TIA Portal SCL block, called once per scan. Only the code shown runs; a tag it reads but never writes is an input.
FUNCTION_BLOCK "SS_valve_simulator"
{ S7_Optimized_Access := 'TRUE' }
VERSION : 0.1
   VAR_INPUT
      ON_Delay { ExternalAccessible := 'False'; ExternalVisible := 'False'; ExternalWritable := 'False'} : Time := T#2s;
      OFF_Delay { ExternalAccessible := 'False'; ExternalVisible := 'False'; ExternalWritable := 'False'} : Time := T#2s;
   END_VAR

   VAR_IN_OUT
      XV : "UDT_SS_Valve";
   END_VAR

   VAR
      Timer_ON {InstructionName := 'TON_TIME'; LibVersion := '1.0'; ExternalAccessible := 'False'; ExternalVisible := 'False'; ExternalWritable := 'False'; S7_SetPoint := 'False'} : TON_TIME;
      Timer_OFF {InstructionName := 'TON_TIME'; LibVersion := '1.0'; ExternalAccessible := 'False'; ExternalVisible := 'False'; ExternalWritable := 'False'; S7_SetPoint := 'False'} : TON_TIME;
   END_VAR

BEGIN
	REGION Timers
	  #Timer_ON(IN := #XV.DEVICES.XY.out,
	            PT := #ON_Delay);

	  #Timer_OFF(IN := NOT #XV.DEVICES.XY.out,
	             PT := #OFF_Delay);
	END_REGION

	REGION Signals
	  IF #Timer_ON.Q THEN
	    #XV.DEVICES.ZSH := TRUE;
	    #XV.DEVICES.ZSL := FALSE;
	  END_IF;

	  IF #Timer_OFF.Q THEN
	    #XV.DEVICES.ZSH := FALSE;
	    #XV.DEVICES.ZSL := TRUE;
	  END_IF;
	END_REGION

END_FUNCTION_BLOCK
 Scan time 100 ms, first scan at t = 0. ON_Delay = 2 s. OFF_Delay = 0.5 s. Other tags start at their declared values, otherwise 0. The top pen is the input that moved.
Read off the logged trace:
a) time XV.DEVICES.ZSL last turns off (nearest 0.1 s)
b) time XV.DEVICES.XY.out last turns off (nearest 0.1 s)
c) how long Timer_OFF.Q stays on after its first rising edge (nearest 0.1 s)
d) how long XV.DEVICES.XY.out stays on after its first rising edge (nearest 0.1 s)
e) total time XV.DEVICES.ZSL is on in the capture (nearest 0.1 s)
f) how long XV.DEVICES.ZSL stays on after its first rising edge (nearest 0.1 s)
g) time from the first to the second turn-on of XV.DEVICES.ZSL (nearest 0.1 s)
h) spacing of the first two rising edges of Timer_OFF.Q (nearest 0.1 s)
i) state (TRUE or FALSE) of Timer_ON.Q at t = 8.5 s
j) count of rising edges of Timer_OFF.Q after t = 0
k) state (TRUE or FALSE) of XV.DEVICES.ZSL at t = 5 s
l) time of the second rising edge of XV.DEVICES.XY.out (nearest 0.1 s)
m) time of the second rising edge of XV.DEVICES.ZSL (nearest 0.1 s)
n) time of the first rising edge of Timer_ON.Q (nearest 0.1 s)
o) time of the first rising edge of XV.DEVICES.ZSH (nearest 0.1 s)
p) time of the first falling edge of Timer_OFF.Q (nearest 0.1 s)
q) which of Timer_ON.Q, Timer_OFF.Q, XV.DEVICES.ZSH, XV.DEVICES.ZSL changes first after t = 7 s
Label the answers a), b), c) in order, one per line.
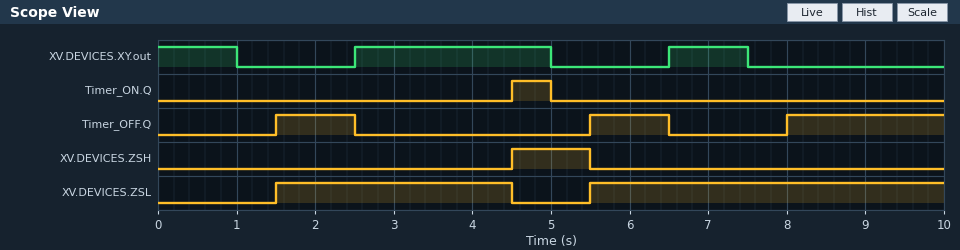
a) 4.5 s
b) 7.5 s
c) 1.0 s
d) 2.5 s
e) 7.5 s
f) 3.0 s
g) 4.0 s
h) 4.0 s
i) FALSE
j) 3
k) FALSE
l) 6.5 s
m) 5.5 s
n) 4.5 s
o) 4.5 s
p) 2.5 s
q) Timer_OFF.Q
